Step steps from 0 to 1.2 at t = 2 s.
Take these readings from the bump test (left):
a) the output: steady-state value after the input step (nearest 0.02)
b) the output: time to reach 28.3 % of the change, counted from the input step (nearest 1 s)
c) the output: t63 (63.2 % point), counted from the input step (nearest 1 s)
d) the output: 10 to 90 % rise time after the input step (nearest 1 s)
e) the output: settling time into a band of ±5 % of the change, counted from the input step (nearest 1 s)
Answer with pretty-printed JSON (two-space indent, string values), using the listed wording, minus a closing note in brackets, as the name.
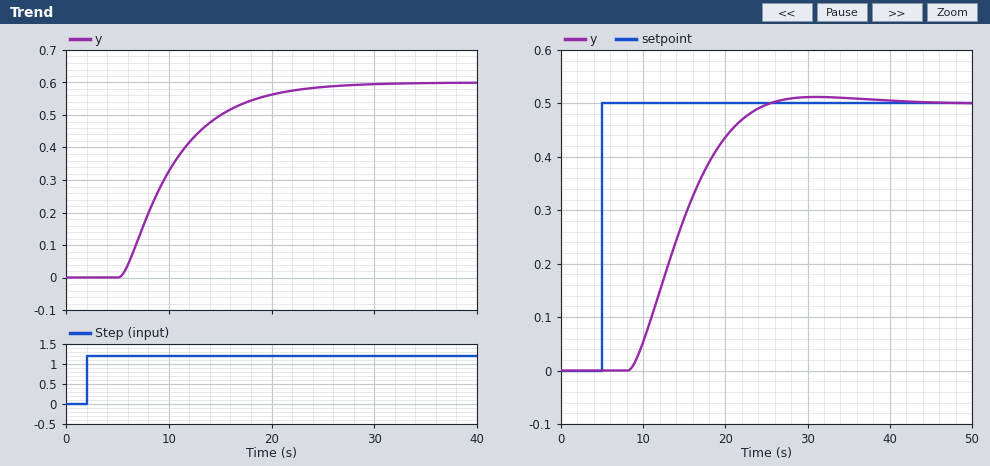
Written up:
{
  "the output: steady-state value after the input step": "0.60",
  "the output: time to reach 28.3 % of the change, counted from the input step": "6 s",
  "the output: t63 (63.2 % point), counted from the input step": "9 s",
  "the output: 10 to 90 % rise time after the input step": "11 s",
  "the output: settling time into a band of ±5 % of the change, counted from the input step": "19 s"
}
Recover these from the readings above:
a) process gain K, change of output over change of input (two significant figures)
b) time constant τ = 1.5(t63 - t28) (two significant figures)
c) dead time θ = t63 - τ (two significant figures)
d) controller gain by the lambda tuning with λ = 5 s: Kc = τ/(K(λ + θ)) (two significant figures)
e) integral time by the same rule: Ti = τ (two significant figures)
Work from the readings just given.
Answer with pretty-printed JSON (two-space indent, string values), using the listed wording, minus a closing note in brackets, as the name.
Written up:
{
  "process gain K, change of output over change of input": "0.50",
  "time constant τ = 1.5(t63 - t28)": "4.5 s",
  "dead time θ = t63 - τ": "4.5 s",
  "controller gain by the lambda tuning with λ = 5 s: Kc = τ/(K(λ + θ))": "0.95",
  "integral time by the same rule: Ti = τ": "4.5 s"
}
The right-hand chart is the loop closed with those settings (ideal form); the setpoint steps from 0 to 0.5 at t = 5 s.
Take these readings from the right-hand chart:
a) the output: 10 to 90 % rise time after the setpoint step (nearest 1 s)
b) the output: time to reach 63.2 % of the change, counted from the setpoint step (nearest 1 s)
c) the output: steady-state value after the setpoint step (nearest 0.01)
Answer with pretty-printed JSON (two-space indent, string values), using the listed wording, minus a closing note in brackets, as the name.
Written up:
{
  "the output: 10 to 90 % rise time after the setpoint step": "11 s",
  "the output: time to reach 63.2 % of the change, counted from the setpoint step": "11 s",
  "the output: steady-state value after the setpoint step": "0.50"
}
